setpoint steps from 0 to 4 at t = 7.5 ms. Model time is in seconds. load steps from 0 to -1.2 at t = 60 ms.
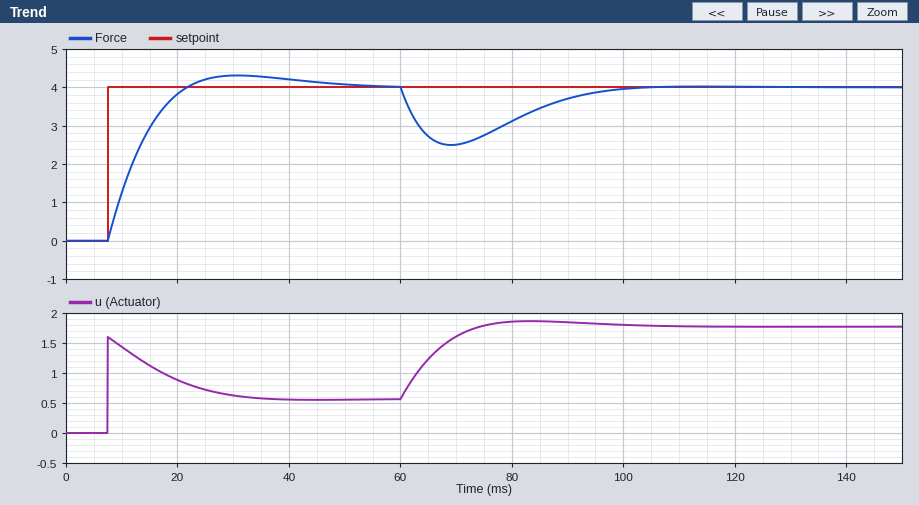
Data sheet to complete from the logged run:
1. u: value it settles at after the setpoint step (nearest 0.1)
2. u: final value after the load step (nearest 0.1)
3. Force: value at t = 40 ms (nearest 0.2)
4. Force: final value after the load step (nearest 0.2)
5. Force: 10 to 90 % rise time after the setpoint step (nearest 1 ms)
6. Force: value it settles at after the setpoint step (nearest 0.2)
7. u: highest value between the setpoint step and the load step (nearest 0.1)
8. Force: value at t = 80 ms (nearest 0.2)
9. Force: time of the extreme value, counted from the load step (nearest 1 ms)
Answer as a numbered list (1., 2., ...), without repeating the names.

1. 0.6
2. 1.8
3. 4.2
4. 4.0
5. 10 ms
6. 4.0
7. 1.6
8. 3.2
9. 9 ms
